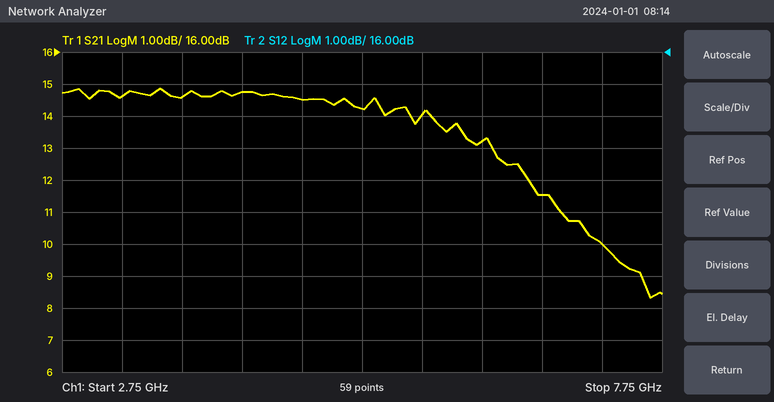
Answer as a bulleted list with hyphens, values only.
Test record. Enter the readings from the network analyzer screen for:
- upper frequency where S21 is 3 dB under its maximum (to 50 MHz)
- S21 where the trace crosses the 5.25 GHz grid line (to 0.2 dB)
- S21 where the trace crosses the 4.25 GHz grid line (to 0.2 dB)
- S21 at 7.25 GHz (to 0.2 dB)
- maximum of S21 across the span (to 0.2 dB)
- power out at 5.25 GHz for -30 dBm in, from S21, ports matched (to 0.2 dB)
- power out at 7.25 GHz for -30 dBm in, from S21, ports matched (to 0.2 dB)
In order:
- 6.65 GHz
- 14.2 dB
- 14.8 dB
- 10.0 dB
- 14.8 dB
- -15.8 dBm
- -20.0 dBm
